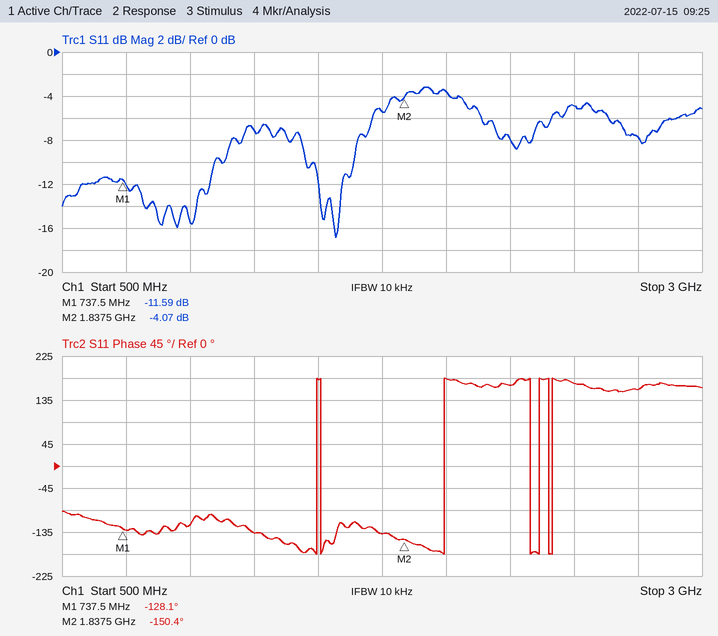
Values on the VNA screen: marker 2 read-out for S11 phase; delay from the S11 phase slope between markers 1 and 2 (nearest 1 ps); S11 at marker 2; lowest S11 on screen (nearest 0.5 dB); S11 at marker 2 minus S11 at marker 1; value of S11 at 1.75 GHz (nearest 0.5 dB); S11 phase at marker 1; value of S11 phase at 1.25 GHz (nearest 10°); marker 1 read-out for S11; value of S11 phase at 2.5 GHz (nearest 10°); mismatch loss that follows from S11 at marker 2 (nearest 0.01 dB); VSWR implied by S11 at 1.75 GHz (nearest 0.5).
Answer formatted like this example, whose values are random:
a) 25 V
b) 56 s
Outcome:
a) -150.4°
b) 56 ps
c) -4.07 dB
d) -17.0 dB
e) 7.52 dB
f) -5.5 dB
g) -128.1°
h) -140°
i) -11.59 dB
j) 170°
k) 2.16 dB
l) 3.5
